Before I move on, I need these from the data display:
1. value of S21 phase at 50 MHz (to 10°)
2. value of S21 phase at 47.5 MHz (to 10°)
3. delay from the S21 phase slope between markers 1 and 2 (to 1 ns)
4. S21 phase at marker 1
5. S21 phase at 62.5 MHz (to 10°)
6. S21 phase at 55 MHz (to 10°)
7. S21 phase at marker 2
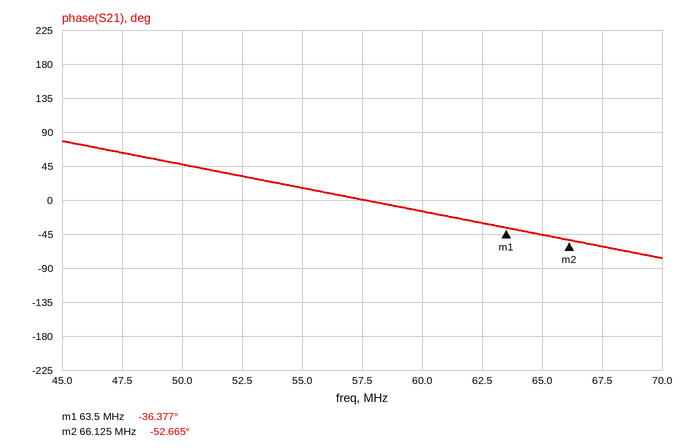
50°
60°
17 ns
-36.377°
-30°
20°
-52.665°
